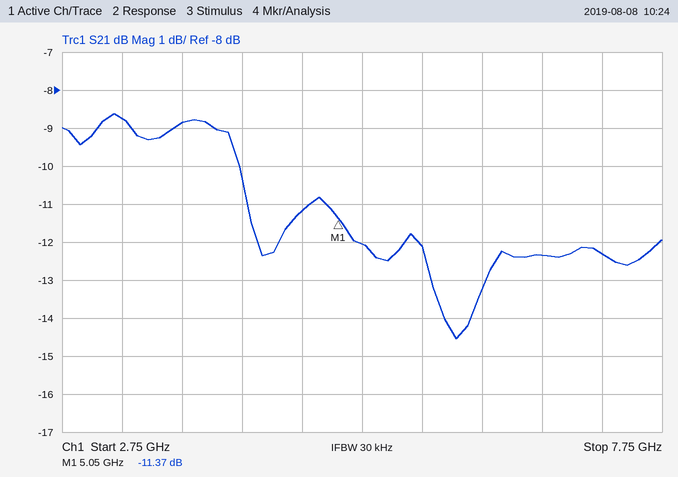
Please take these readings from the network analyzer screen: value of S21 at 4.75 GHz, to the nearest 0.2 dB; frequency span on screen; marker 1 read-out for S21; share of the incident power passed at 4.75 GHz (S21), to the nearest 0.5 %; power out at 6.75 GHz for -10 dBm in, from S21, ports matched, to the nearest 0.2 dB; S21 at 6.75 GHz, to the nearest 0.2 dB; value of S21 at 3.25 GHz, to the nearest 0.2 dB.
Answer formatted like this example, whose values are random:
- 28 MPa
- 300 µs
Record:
- -11.2 dB
- 5 GHz
- -11.37 dB
- 7.5 %
- -22.4 dBm
- -12.4 dB
- -8.8 dB
